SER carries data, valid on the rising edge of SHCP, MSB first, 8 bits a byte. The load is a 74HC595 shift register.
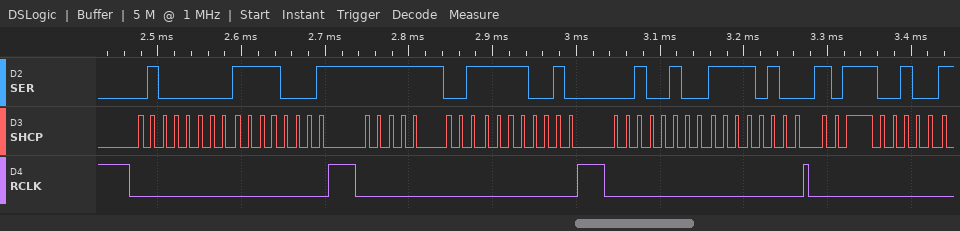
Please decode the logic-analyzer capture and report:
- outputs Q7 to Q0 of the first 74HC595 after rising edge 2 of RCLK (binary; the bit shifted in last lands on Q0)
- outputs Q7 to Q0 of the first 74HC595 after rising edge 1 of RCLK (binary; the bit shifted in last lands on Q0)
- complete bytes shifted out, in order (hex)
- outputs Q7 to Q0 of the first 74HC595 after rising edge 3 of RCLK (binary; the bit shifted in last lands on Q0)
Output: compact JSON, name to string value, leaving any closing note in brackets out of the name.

{"outputs Q7 to Q0 of the first 74HC595 after rising edge 2 of RCLK": "11110010", "outputs Q7 to Q0 of the first 74HC595 after rising edge 1 of RCLK": "11110001", "complete bytes shifted out, in order": "0x40 0xF1 0xF9 0xF2 0x24 0xF4 0xA4", "outputs Q7 to Q0 of the first 74HC595 after rising edge 3 of RCLK": "11110100"}
